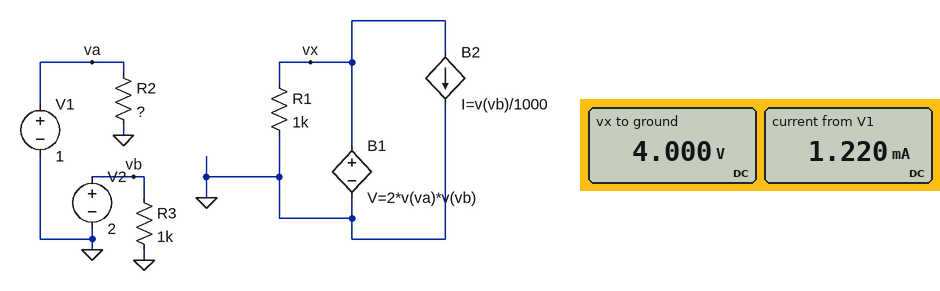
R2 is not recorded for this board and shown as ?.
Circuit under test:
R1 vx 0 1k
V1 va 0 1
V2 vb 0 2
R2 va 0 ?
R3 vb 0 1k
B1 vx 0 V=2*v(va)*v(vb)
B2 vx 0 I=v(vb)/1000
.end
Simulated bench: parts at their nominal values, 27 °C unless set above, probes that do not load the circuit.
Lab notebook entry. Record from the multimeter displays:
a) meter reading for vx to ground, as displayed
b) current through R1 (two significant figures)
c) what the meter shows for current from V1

4.000 V
4.0 mA
1.220 mA
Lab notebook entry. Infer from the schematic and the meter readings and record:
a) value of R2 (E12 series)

820 Ω
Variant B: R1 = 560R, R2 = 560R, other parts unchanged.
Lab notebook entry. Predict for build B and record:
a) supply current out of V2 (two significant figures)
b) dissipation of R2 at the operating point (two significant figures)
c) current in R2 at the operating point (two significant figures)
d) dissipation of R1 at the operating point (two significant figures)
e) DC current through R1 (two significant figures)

2.0 mA
1.8 mW
1.8 mA
29 mW
7.1 mA
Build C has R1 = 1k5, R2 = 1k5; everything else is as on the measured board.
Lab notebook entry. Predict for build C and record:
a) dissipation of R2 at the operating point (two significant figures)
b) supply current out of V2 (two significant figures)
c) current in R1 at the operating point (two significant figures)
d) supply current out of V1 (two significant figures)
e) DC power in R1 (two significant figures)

670 µW
2.0 mA
2.7 mA
670 µA
11 mW
